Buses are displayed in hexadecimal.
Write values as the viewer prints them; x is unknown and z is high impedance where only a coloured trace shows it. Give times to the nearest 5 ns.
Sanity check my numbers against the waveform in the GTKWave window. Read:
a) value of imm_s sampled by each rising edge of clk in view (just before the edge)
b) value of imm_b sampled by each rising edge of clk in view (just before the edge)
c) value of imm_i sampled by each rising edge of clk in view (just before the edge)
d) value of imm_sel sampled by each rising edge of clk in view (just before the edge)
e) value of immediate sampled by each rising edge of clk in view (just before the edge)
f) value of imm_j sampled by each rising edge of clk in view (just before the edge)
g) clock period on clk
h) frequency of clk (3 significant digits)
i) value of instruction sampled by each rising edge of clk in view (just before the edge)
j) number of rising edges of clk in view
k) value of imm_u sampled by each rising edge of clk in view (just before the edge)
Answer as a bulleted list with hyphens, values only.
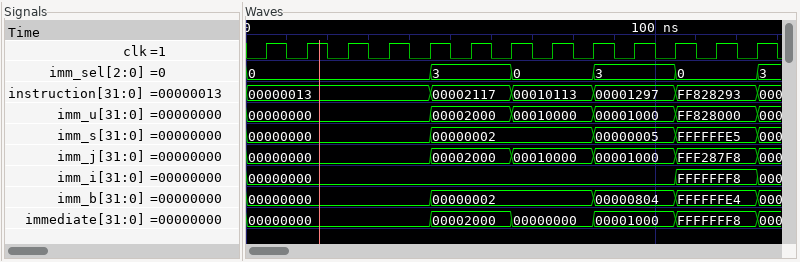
- 00000000, 00000000, 00000000, 00000000, 00000000, 00000002, 00000002, 00000002, 00000002, 00000005, 00000005, FFFFFFE5, FFFFFFE5
- 00000000, 00000000, 00000000, 00000000, 00000000, 00000002, 00000002, 00000002, 00000002, 00000804, 00000804, FFFFFFE4, FFFFFFE4
- 00000000, 00000000, 00000000, 00000000, 00000000, 00000000, 00000000, 00000000, 00000000, 00000000, 00000000, FFFFFFF8, FFFFFFF8
- 0, 0, 0, 0, 0, 3, 3, 0, 0, 3, 3, 0, 0
- 00000000, 00000000, 00000000, 00000000, 00000000, 00002000, 00002000, 00000000, 00000000, 00001000, 00001000, FFFFFFF8, FFFFFFF8
- 00000000, 00000000, 00000000, 00000000, 00000000, 00002000, 00002000, 00010000, 00010000, 00001000, 00001000, FFF287F8, FFF287F8
- 10 ns
- 100 MHz
- 00000013, 00000013, 00000013, 00000013, 00000013, 00002117, 00002117, 00010113, 00010113, 00001297, 00001297, FF828293, FF828293
- 13
- 00000000, 00000000, 00000000, 00000000, 00000000, 00002000, 00002000, 00010000, 00010000, 00001000, 00001000, FF828000, FF828000
